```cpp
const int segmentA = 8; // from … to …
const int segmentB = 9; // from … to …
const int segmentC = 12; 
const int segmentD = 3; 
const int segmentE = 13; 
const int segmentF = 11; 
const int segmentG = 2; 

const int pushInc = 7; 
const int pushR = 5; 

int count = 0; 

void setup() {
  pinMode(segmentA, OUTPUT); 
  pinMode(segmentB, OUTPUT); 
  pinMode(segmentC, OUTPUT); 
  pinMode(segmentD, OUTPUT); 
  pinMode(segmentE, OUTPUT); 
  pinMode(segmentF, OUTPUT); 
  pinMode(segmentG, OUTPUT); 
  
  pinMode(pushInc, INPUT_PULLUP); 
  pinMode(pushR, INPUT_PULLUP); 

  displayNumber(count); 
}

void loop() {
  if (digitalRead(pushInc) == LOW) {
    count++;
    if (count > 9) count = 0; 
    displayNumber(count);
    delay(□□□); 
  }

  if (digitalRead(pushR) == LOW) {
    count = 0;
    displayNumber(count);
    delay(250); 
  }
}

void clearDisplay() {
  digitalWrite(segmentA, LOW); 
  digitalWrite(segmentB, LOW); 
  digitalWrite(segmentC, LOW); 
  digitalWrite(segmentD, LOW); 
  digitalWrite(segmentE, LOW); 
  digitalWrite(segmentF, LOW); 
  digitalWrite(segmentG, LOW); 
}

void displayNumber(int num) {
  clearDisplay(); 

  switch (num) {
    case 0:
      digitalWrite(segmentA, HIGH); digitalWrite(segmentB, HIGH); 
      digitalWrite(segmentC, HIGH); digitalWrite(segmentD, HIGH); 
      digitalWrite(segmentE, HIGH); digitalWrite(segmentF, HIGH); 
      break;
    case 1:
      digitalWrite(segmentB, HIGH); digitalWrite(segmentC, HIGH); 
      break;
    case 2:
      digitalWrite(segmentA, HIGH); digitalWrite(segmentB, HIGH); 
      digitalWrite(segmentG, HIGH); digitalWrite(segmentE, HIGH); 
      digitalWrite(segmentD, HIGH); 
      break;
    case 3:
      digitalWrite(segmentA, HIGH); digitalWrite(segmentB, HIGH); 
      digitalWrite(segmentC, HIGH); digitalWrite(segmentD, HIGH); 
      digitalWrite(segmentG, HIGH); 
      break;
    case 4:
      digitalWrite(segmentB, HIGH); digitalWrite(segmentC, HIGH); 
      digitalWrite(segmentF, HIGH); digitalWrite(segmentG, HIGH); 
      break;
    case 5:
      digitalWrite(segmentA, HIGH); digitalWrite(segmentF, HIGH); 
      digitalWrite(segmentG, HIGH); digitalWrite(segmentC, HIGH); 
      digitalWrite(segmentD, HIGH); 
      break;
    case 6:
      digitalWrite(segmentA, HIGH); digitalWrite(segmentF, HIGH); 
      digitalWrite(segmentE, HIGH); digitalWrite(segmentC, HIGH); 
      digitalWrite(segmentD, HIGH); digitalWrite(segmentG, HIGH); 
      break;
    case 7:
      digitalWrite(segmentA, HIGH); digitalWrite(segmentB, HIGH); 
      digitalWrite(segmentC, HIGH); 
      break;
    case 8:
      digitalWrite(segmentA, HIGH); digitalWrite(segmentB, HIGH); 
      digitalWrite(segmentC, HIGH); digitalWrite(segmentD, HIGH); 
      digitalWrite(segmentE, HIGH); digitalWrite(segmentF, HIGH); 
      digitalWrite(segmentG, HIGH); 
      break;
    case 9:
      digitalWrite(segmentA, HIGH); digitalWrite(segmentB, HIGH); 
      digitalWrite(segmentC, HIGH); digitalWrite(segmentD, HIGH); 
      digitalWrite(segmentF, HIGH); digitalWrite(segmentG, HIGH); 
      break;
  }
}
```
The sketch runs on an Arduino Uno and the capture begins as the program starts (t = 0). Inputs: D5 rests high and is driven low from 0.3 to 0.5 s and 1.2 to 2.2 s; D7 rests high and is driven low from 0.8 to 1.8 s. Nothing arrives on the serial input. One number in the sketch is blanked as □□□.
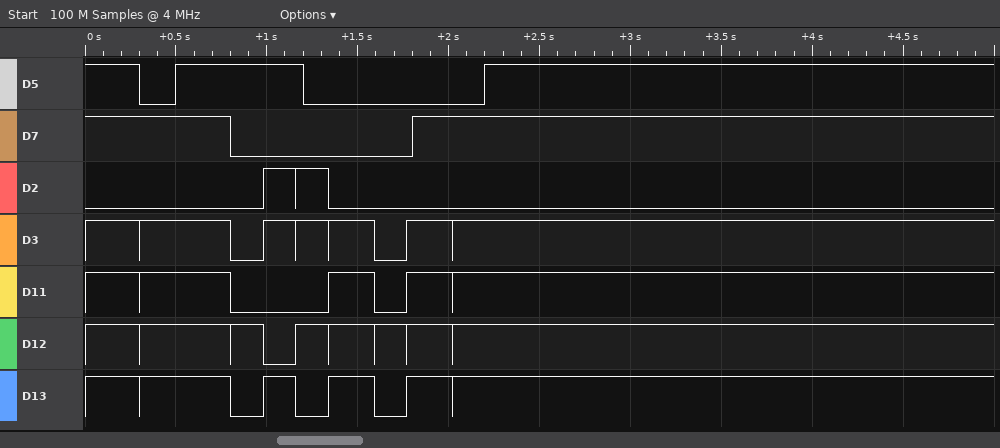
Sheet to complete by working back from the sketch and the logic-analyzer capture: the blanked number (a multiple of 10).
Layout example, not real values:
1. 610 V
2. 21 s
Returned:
1. 180
